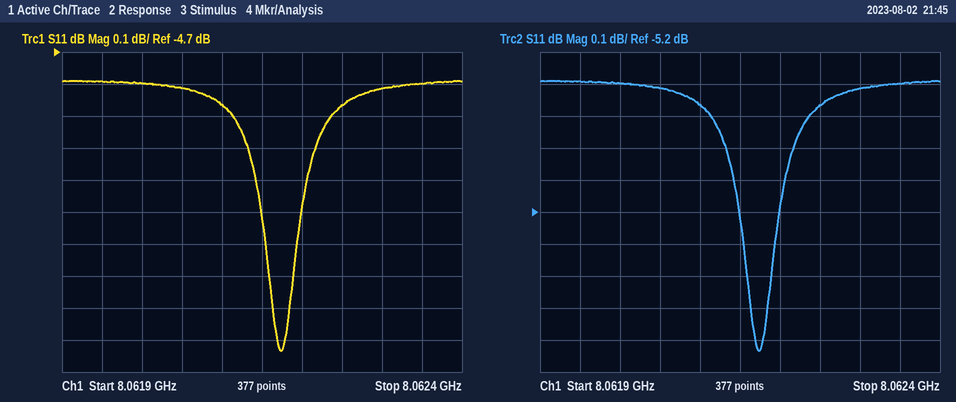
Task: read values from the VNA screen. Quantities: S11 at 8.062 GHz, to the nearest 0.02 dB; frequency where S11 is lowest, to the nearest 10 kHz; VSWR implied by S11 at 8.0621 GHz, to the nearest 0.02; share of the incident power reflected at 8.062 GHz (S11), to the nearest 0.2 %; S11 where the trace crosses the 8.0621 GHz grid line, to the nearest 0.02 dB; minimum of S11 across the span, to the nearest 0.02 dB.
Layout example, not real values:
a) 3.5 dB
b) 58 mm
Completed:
a) -4.80 dB
b) 8.06217 GHz
c) 3.66
d) 33.2 %
e) -4.86 dB
f) -5.64 dB
